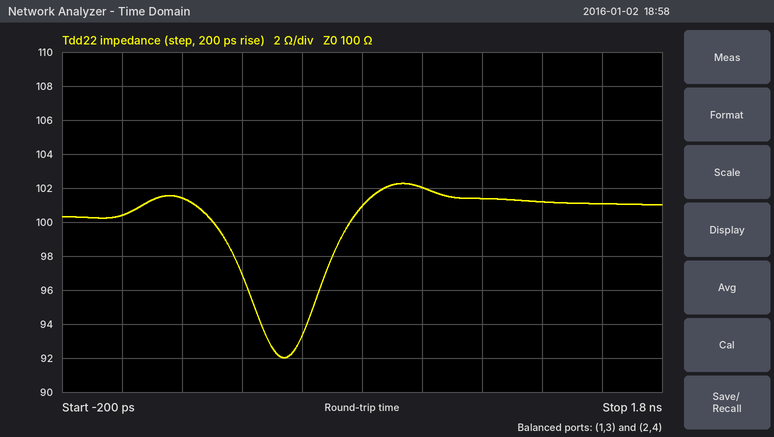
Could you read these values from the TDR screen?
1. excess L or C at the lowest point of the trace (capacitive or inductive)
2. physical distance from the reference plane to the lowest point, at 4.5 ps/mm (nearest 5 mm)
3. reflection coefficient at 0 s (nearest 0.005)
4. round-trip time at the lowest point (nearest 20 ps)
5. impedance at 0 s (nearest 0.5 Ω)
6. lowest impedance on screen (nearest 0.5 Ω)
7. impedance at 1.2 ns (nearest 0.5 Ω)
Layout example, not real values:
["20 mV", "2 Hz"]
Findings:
["capacitive", "60 mm", "0.000", "540 ps", "100.5 Ω", "92.0 Ω", "101.5 Ω"]
